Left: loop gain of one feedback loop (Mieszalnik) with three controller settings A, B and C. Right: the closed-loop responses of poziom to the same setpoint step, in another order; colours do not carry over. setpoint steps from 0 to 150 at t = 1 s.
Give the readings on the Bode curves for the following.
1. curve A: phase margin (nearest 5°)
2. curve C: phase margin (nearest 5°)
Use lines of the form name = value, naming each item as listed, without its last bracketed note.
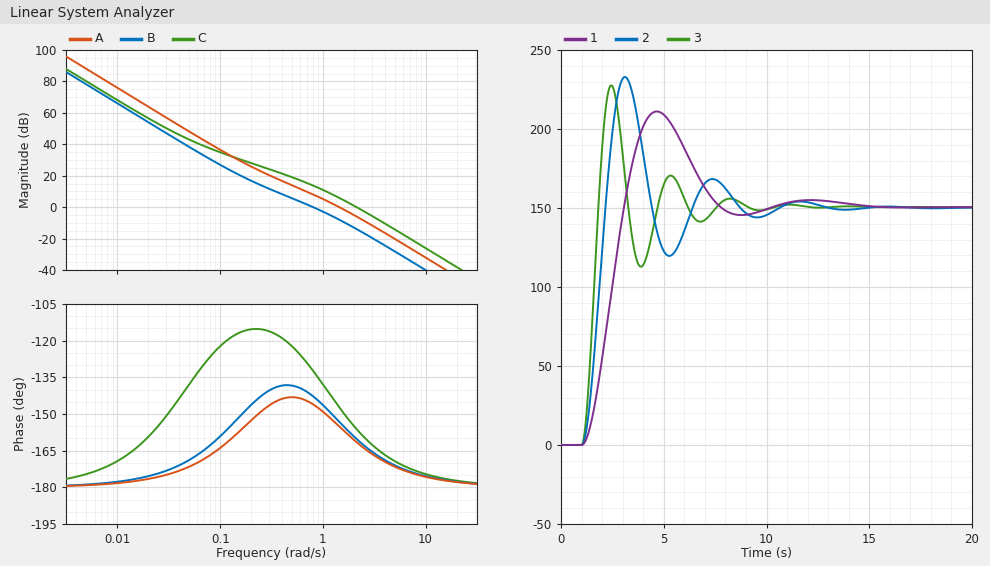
curve A: phase margin = 25°
curve C: phase margin = 25°
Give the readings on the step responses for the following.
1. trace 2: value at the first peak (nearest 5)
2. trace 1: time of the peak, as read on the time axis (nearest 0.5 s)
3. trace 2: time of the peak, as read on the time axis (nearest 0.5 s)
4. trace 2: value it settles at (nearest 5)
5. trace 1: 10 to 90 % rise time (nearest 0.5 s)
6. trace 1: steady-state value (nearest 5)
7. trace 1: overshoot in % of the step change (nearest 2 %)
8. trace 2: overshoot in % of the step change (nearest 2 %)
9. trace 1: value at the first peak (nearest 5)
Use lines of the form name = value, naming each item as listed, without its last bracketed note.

trace 2: value at the first peak = 235
trace 1: time of the peak, as read on the time axis = 4.5 s
trace 2: time of the peak, as read on the time axis = 3.0 s
trace 2: value it settles at = 150
trace 1: 10 to 90 % rise time = 1.5 s
trace 1: steady-state value = 150
trace 1: overshoot in % of the step change = 40 %
trace 2: overshoot in % of the step change = 56 %
trace 1: value at the first peak = 210
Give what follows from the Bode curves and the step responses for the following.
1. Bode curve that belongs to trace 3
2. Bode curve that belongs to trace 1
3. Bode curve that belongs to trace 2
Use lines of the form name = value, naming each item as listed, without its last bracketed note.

Bode curve that belongs to trace 3 = C
Bode curve that belongs to trace 1 = B
Bode curve that belongs to trace 2 = A
